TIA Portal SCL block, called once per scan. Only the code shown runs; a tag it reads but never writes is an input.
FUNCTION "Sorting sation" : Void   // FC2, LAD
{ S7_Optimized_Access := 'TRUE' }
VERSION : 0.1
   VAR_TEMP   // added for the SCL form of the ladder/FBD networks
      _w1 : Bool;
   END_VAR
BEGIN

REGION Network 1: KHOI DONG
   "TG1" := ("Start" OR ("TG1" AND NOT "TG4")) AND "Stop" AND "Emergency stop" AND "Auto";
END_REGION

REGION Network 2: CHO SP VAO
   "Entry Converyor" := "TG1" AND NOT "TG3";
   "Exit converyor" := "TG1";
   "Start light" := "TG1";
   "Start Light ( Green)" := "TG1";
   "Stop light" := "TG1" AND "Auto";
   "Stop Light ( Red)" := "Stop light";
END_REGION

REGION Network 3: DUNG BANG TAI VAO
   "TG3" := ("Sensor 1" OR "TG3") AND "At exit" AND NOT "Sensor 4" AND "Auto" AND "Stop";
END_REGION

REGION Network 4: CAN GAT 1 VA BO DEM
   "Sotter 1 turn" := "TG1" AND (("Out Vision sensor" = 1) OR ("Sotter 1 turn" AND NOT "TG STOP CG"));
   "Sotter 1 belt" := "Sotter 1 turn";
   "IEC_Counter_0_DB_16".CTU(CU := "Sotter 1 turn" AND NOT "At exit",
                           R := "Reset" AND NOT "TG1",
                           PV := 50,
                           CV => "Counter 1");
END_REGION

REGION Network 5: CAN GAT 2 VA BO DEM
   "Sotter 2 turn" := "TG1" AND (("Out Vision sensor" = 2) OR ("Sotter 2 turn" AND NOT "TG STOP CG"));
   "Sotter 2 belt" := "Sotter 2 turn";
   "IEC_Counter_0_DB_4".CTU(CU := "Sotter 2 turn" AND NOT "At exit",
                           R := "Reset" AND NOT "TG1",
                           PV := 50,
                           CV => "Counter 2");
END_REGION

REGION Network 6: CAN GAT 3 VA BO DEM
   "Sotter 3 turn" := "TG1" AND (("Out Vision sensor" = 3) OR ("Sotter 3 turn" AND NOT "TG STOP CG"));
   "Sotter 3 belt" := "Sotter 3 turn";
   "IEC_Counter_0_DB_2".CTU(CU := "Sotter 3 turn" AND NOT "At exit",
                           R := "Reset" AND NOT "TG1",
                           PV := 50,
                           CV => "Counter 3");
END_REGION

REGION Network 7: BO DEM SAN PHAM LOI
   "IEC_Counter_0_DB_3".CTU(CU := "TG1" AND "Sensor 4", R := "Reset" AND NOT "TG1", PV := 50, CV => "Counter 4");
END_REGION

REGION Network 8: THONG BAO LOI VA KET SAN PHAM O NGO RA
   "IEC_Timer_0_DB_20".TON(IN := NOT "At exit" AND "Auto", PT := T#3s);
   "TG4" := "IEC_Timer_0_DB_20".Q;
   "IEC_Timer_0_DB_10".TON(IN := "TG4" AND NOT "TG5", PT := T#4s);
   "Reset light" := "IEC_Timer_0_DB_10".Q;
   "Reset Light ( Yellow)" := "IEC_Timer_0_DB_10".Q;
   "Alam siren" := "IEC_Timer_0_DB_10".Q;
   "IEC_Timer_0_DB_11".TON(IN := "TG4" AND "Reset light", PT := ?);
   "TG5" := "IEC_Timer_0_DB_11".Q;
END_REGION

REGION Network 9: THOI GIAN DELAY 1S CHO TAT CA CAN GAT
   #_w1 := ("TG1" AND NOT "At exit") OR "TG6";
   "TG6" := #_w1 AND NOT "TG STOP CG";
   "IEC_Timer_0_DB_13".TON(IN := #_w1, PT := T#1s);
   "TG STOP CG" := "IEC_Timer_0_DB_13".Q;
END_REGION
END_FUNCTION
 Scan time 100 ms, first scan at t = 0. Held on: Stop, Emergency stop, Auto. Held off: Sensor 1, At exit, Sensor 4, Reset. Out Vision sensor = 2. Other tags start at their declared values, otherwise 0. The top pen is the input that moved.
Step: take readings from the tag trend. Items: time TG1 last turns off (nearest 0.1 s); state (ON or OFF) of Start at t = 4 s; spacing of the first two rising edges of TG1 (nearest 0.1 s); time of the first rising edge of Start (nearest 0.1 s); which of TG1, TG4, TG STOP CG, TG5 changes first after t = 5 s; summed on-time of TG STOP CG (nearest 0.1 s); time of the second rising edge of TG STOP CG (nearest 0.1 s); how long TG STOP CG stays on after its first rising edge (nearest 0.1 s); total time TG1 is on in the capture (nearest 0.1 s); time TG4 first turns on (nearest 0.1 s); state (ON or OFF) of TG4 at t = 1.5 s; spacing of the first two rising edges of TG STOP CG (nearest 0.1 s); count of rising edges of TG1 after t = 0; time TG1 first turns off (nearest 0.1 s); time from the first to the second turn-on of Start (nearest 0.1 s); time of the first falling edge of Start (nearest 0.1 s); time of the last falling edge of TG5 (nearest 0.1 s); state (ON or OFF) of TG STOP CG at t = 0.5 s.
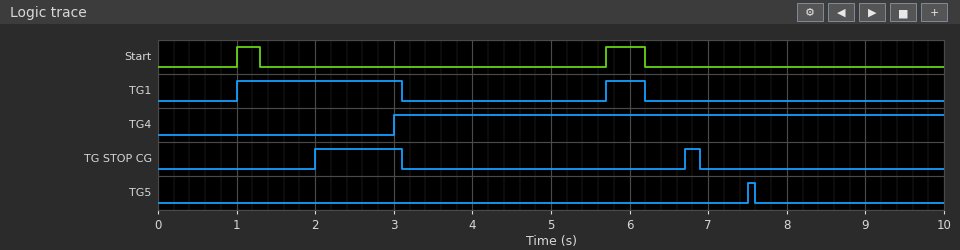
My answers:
6.2 s
OFF
4.7 s
1.0 s
TG1
1.3 s
6.7 s
1.1 s
2.6 s
3.0 s
OFF
4.7 s
2
3.1 s
4.7 s
1.3 s
7.6 s
OFF
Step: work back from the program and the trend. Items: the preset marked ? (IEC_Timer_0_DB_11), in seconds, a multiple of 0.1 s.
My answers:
0.5 s
